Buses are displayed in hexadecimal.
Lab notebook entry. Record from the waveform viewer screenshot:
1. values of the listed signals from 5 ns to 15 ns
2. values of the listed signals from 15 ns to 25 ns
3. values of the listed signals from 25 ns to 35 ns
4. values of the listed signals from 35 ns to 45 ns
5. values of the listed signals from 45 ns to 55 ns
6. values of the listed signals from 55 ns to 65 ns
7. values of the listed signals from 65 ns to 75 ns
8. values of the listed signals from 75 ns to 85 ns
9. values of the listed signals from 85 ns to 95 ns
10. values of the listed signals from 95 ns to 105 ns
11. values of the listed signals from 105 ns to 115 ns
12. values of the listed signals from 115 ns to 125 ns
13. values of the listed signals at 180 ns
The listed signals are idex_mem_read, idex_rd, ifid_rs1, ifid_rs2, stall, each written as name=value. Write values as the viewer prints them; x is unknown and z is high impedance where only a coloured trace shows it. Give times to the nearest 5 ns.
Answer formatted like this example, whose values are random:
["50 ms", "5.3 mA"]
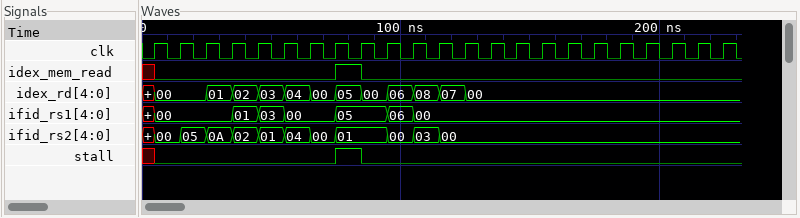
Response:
["idex_mem_read=0, idex_rd=00, ifid_rs1=00, ifid_rs2=00, stall=0", "idex_mem_read=0, idex_rd=00, ifid_rs1=00, ifid_rs2=05, stall=0", "idex_mem_read=0, idex_rd=01, ifid_rs1=00, ifid_rs2=0A, stall=0", "idex_mem_read=0, idex_rd=02, ifid_rs1=01, ifid_rs2=02, stall=0", "idex_mem_read=0, idex_rd=03, ifid_rs1=03, ifid_rs2=01, stall=0", "idex_mem_read=0, idex_rd=04, ifid_rs1=00, ifid_rs2=04, stall=0", "idex_mem_read=0, idex_rd=00, ifid_rs1=00, ifid_rs2=00, stall=0", "idex_mem_read=1, idex_rd=05, ifid_rs1=05, ifid_rs2=01, stall=1", "idex_mem_read=0, idex_rd=00, ifid_rs1=05, ifid_rs2=01, stall=0", "idex_mem_read=0, idex_rd=06, ifid_rs1=06, ifid_rs2=00, stall=0", "idex_mem_read=0, idex_rd=08, ifid_rs1=00, ifid_rs2=03, stall=0", "idex_mem_read=0, idex_rd=07, ifid_rs1=00, ifid_rs2=00, stall=0", "idex_mem_read=0, idex_rd=00, ifid_rs1=00, ifid_rs2=00, stall=0"]
